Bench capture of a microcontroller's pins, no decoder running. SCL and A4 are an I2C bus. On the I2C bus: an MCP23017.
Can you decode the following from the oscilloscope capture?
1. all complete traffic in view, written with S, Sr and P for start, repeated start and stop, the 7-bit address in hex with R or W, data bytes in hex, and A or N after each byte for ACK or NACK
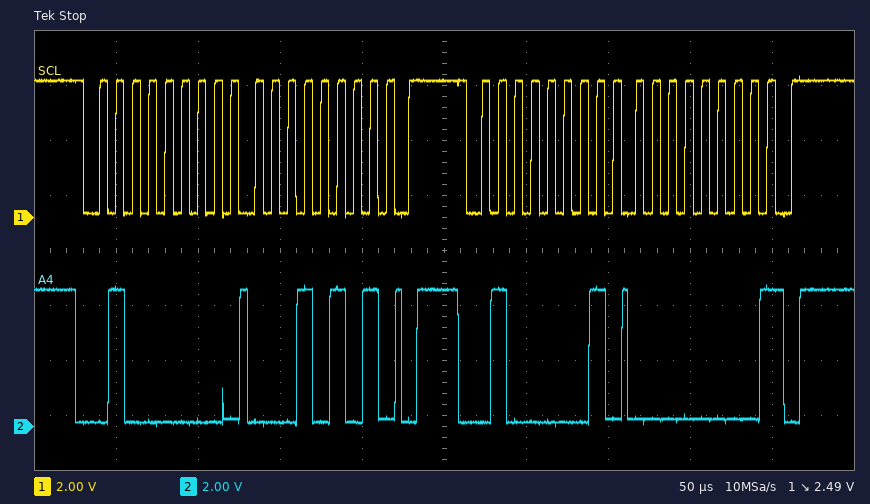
S 20W A 15 A P S 20R A 00 N P
